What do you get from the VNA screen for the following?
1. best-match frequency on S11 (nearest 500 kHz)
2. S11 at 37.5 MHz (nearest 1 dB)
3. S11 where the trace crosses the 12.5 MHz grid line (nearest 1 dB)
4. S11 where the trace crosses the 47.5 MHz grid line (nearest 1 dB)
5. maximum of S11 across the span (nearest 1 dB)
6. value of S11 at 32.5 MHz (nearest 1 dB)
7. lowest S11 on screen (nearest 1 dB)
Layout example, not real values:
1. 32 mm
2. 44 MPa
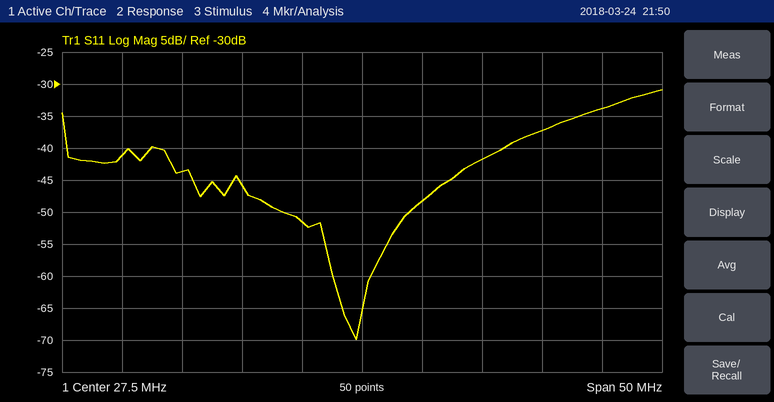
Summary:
1. 27.0 MHz
2. -42 dB
3. -44 dB
4. -34 dB
5. -31 dB
6. -48 dB
7. -70 dB
